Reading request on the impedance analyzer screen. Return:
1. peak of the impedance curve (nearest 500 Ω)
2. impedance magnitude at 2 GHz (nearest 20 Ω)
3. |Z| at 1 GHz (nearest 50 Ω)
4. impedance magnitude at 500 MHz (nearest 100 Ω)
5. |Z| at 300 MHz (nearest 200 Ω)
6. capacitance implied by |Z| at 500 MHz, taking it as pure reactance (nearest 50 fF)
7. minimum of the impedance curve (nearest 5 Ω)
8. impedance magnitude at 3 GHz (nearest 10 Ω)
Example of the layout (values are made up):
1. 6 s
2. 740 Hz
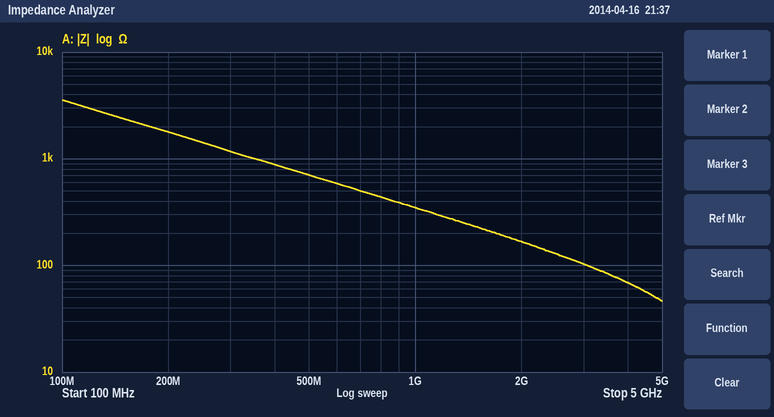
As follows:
1. 3.5 kΩ
2. 160 Ω
3. 350 Ω
4. 700 Ω
5. 1.2 kΩ
6. 450 fF
7. 45 Ω
8. 100 Ω
